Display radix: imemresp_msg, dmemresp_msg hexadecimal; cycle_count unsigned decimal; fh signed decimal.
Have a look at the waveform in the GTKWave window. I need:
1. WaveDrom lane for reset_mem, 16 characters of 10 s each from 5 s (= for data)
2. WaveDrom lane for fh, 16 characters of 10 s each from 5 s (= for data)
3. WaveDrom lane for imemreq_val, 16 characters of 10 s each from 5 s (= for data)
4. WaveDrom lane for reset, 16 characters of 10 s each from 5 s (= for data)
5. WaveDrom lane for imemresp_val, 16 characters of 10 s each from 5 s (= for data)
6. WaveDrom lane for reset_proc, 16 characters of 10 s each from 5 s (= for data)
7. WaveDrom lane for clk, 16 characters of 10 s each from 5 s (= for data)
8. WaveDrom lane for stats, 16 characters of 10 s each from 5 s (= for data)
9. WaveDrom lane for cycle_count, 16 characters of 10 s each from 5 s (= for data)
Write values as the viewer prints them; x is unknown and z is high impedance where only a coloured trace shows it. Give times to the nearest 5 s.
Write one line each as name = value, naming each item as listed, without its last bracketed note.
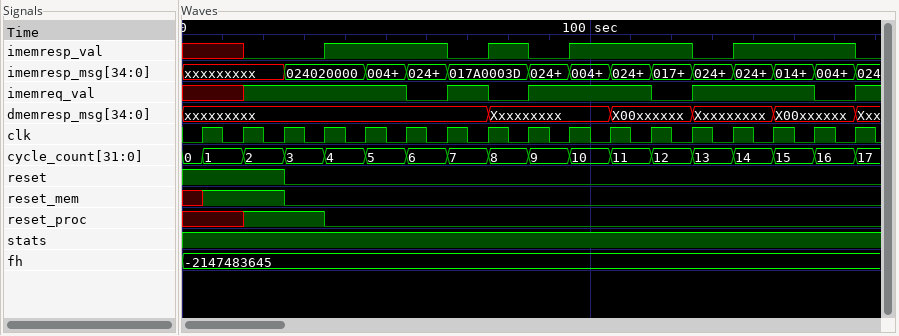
WaveDrom lane for reset_mem, 16 characters of 10 s each from 5 s = {name: 'reset_mem', wave: '1.0.............'}
WaveDrom lane for fh, 16 characters of 10 s each from 5 s = {name: 'fh', wave: '=...............', data: '-2147483645'}
WaveDrom lane for imemreq_val, 16 characters of 10 s each from 5 s = {name: 'imemreq_val', wave: 'x1...0101..01..0'}
WaveDrom lane for reset, 16 characters of 10 s each from 5 s = {name: 'reset', wave: '1.0.............'}
WaveDrom lane for imemresp_val, 16 characters of 10 s each from 5 s = {name: 'imemresp_val', wave: 'x0.1..0101..01..'}
WaveDrom lane for reset_proc, 16 characters of 10 s each from 5 s = {name: 'reset_proc', wave: 'x1.0............'}
WaveDrom lane for clk, 16 characters of 10 s each from 5 s = {name: 'clk', wave: 'p...............'}
WaveDrom lane for stats, 16 characters of 10 s each from 5 s = {name: 'stats', wave: '1...............'}
WaveDrom lane for cycle_count, 16 characters of 10 s each from 5 s = {name: 'cycle_count', wave: '================', data: '1 2 3 4 5 6 7 8 9 10 11 12 13 14 15 16'}
